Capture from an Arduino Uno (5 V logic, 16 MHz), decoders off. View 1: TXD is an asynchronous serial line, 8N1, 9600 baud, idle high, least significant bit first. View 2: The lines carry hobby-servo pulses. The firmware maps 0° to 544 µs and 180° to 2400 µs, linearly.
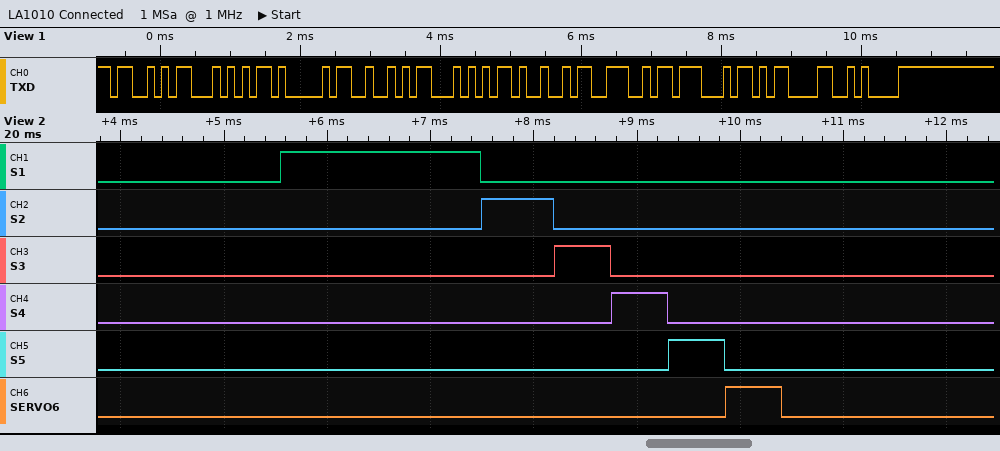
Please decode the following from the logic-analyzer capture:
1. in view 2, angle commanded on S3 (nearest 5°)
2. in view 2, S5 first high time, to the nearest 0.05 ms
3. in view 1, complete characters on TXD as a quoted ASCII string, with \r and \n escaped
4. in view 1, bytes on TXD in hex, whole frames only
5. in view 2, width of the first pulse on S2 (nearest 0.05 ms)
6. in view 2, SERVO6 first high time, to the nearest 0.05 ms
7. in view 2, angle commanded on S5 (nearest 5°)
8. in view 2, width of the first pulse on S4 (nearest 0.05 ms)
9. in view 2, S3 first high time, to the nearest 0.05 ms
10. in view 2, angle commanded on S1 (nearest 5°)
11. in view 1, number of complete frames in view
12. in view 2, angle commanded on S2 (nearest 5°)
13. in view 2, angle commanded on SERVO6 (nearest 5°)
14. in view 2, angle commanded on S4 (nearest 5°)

0°
0.55 ms
"STARTING\r\n"
0x53 0x54 0x41 0x52 0x54 0x49 0x4E 0x47 0x0D 0x0A
0.70 ms
0.55 ms
0°
0.55 ms
0.55 ms
135°
10
15°
0°
0°
